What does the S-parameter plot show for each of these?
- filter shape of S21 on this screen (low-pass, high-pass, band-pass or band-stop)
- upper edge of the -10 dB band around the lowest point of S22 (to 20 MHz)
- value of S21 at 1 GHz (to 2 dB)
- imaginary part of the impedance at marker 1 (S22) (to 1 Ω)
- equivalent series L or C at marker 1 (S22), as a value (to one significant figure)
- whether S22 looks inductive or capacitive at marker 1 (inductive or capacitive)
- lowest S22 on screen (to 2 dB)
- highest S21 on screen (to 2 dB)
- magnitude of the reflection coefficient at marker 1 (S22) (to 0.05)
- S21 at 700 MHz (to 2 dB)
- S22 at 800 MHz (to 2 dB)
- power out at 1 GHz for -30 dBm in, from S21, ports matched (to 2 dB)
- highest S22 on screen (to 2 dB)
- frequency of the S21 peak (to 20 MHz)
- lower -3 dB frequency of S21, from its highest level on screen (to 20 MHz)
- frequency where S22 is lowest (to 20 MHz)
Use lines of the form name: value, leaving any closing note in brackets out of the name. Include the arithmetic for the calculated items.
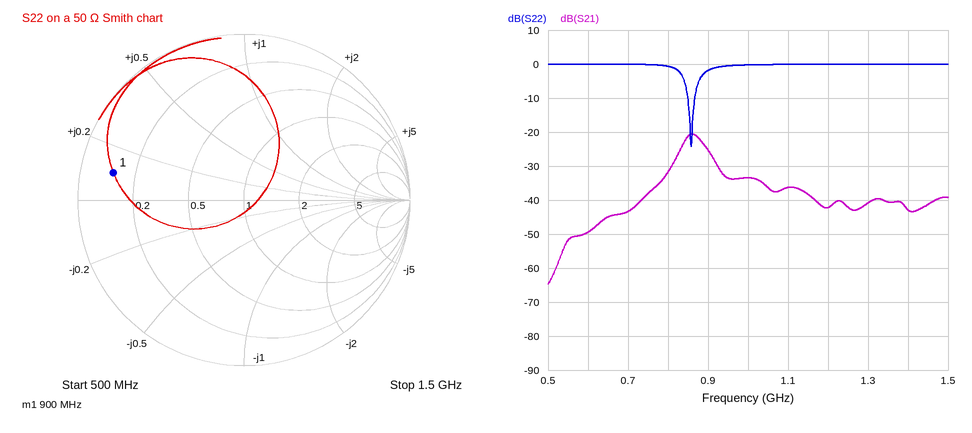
filter shape of S21 on this screen: band-pass
upper edge of the -10 dB band around the lowest point of S22: 860 MHz
value of S21 at 1 GHz: -34 dB
imaginary part of the impedance at marker 1 (S22): +5 Ω
equivalent series L or C at marker 1 (S22), as a value: L = 5 Ω/(2π × 900 MHz) ≈ 884 pH, so 900 pH to one significant figure
whether S22 looks inductive or capacitive at marker 1: inductive
lowest S22 on screen: -24 dB
highest S21 on screen: -20 dB
magnitude of the reflection coefficient at marker 1 (S22): 0.80
S21 at 700 MHz: -44 dB
S22 at 800 MHz: 0 dB
power out at 1 GHz for -30 dBm in, from S21, ports matched: -30 dBm + (-34 dB) = -64 dBm
highest S22 on screen: 0 dB
frequency of the S21 peak: 860 MHz
lower -3 dB frequency of S21, from its highest level on screen: 840 MHz
frequency where S22 is lowest: 860 MHz
